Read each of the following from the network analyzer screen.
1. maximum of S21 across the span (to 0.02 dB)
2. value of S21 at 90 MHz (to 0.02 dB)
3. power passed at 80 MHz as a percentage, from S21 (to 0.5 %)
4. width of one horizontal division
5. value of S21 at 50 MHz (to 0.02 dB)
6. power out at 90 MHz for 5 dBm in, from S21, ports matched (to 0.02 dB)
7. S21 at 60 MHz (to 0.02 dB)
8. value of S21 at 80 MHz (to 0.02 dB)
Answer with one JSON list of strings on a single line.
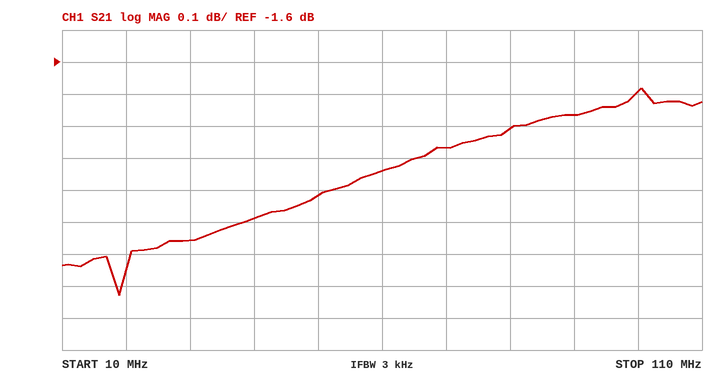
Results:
["-1.68 dB", "-1.76 dB", "66.0 %", "10 MHz", "-2.02 dB", "3.24 dBm", "-1.94 dB", "-1.80 dB"]
